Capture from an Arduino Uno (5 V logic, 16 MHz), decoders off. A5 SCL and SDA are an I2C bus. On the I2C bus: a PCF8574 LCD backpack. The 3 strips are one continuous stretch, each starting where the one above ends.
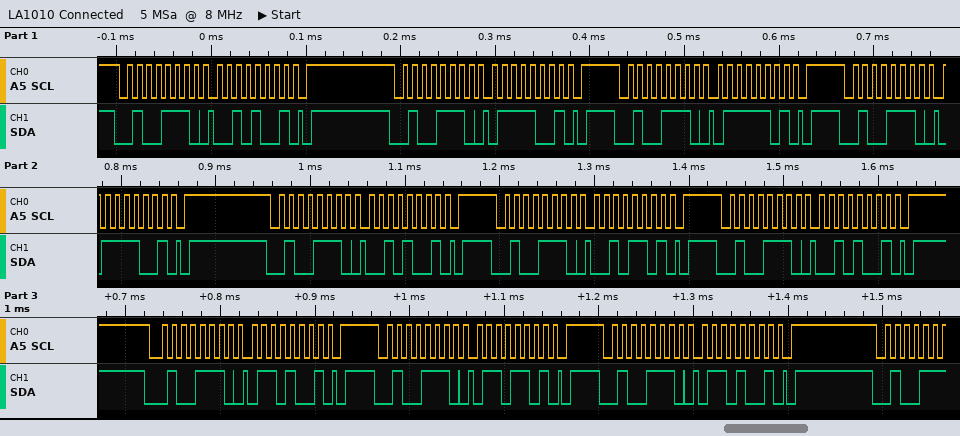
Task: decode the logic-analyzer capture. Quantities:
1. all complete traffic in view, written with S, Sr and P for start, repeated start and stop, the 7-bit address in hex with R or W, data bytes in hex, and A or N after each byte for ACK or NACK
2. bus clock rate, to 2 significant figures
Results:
S 27W A 29 A P S 27W A 79 A P S 27W A 7D A P S 27W A 79 A P S 27W A 29 A P S 27W A 2D A P S 27W A 29 A P S 27W A 69 A P S 27W A 6D A P S 27W A 69 A P
100 kHz
